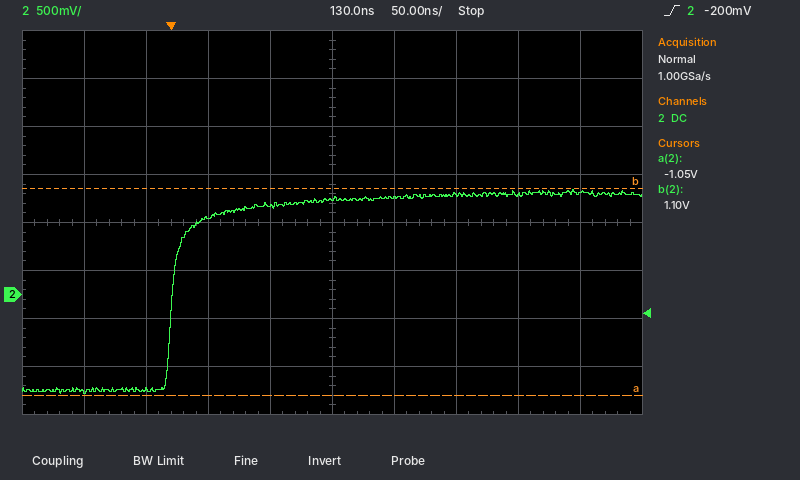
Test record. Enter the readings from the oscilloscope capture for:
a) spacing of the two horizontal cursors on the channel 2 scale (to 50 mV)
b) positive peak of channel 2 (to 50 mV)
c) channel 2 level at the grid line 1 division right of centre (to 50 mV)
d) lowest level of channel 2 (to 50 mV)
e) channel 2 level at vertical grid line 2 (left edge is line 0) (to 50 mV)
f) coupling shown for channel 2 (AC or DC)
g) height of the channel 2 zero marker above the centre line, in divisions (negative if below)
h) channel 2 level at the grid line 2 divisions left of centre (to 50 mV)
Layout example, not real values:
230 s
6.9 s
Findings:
2.15 V
1.10 V
1.00 V
-1.05 V
-1.00 V
DC
-1.5 div
800 mV
